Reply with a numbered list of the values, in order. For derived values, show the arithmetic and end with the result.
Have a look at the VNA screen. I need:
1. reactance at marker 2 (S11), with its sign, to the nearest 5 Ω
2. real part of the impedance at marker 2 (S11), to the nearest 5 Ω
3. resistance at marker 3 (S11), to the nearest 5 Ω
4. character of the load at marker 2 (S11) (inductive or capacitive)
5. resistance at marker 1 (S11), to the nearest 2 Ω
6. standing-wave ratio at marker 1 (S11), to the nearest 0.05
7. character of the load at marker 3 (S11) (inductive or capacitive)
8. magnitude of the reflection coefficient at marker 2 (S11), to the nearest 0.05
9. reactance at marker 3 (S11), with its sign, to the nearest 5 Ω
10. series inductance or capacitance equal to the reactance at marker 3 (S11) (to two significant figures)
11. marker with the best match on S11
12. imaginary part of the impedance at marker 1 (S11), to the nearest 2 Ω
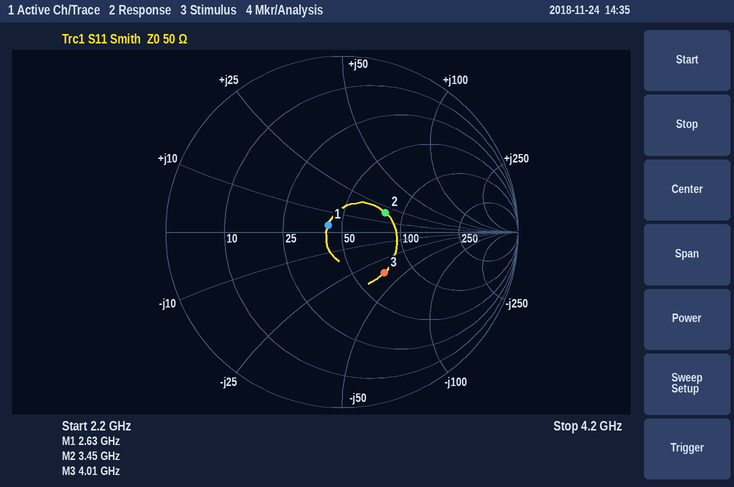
1. +20 Ω
2. 80 Ω
3. 70 Ω
4. inductive
5. 42 Ω
6. 1.20
7. capacitive
8. 0.25
9. -35 Ω
10. C = 1/(2π × 4.01 GHz × 35 Ω) ≈ 1.1 pF
11. marker 1
12. +4 Ω
